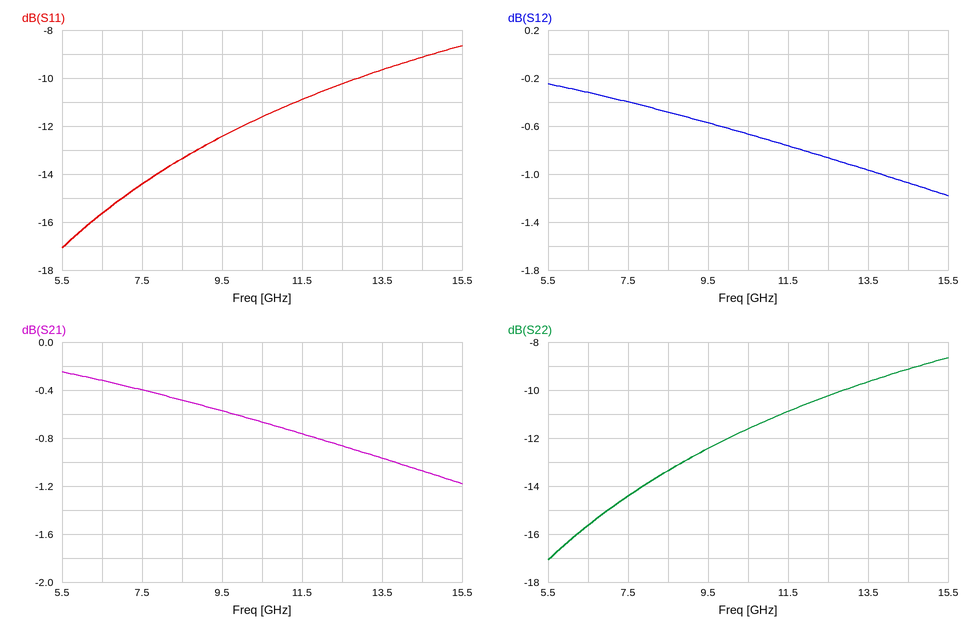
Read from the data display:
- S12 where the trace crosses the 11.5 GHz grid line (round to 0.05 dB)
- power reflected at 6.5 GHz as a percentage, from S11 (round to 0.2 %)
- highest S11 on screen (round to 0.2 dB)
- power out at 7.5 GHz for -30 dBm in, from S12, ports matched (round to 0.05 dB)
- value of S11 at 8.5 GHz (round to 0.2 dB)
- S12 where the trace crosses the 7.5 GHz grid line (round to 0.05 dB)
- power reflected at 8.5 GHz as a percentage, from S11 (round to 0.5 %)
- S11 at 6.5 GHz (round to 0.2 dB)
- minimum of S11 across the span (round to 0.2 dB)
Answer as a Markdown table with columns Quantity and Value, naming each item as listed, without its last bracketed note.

| Quantity | Value |
|---|---|
| S12 where the trace crosses the 11.5 GHz grid line | -0.75 dB |
| power reflected at 6.5 GHz as a percentage, from S11 | 2.8 % |
| highest S11 on screen | -8.6 dB |
| power out at 7.5 GHz for -30 dBm in, from S12, ports matched | -30.40 dBm |
| value of S11 at 8.5 GHz | -13.4 dB |
| S12 where the trace crosses the 7.5 GHz grid line | -0.40 dB |
| power reflected at 8.5 GHz as a percentage, from S11 | 4.5 % |
| S11 at 6.5 GHz | -15.6 dB |
| minimum of S11 across the span | -17.0 dB |
